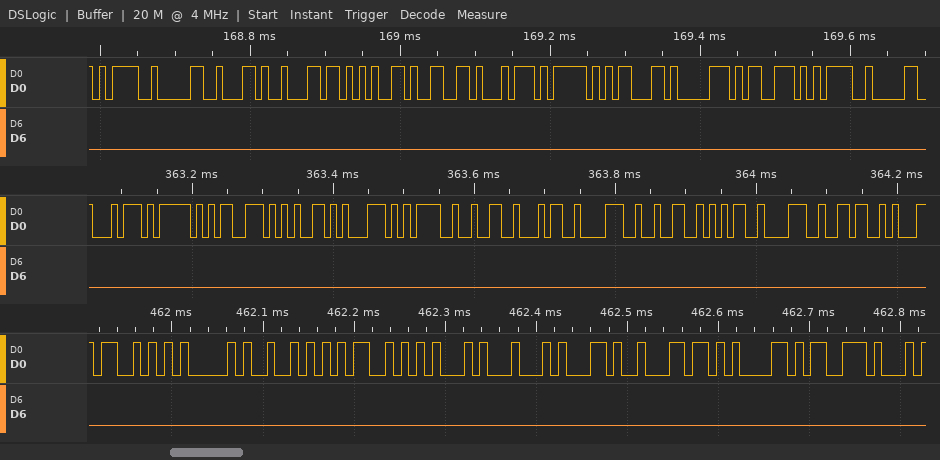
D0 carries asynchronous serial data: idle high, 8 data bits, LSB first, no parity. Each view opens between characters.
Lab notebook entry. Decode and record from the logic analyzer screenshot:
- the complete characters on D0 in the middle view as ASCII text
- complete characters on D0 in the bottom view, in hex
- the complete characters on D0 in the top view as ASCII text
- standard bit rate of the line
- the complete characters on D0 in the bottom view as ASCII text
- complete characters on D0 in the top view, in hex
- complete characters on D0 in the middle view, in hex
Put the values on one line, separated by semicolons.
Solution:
"t_seq=2482586"; 53, 41, 52, 4D, 45, 44, 2C, 6C, 61, 73; "=0,left_cps="; 115200 baud; "SARMED,las"; 3D, 30, 2C, 6C, 65, 66, 74, 5F, 63, 70, 73, 3D; 74, 5F, 73, 65, 71, 3D, 32, 34, 38, 32, 35, 38, 36
